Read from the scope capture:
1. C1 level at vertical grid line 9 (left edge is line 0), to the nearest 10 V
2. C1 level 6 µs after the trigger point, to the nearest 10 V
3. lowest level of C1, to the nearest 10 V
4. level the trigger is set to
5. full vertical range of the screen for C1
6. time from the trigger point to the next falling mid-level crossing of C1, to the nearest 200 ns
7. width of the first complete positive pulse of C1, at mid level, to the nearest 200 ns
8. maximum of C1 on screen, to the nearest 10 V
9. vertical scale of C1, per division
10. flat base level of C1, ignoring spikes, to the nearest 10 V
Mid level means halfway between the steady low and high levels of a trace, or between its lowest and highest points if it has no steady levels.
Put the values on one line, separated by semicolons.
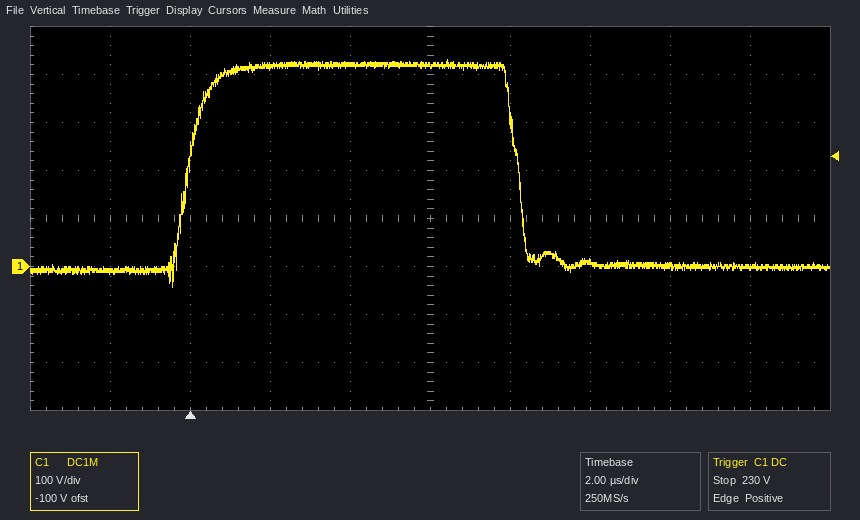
0 V; 420 V; -40 V; 230 V; 800 V; 8.2 µs; 8.2 µs; 430 V; 100 V; 0 V
